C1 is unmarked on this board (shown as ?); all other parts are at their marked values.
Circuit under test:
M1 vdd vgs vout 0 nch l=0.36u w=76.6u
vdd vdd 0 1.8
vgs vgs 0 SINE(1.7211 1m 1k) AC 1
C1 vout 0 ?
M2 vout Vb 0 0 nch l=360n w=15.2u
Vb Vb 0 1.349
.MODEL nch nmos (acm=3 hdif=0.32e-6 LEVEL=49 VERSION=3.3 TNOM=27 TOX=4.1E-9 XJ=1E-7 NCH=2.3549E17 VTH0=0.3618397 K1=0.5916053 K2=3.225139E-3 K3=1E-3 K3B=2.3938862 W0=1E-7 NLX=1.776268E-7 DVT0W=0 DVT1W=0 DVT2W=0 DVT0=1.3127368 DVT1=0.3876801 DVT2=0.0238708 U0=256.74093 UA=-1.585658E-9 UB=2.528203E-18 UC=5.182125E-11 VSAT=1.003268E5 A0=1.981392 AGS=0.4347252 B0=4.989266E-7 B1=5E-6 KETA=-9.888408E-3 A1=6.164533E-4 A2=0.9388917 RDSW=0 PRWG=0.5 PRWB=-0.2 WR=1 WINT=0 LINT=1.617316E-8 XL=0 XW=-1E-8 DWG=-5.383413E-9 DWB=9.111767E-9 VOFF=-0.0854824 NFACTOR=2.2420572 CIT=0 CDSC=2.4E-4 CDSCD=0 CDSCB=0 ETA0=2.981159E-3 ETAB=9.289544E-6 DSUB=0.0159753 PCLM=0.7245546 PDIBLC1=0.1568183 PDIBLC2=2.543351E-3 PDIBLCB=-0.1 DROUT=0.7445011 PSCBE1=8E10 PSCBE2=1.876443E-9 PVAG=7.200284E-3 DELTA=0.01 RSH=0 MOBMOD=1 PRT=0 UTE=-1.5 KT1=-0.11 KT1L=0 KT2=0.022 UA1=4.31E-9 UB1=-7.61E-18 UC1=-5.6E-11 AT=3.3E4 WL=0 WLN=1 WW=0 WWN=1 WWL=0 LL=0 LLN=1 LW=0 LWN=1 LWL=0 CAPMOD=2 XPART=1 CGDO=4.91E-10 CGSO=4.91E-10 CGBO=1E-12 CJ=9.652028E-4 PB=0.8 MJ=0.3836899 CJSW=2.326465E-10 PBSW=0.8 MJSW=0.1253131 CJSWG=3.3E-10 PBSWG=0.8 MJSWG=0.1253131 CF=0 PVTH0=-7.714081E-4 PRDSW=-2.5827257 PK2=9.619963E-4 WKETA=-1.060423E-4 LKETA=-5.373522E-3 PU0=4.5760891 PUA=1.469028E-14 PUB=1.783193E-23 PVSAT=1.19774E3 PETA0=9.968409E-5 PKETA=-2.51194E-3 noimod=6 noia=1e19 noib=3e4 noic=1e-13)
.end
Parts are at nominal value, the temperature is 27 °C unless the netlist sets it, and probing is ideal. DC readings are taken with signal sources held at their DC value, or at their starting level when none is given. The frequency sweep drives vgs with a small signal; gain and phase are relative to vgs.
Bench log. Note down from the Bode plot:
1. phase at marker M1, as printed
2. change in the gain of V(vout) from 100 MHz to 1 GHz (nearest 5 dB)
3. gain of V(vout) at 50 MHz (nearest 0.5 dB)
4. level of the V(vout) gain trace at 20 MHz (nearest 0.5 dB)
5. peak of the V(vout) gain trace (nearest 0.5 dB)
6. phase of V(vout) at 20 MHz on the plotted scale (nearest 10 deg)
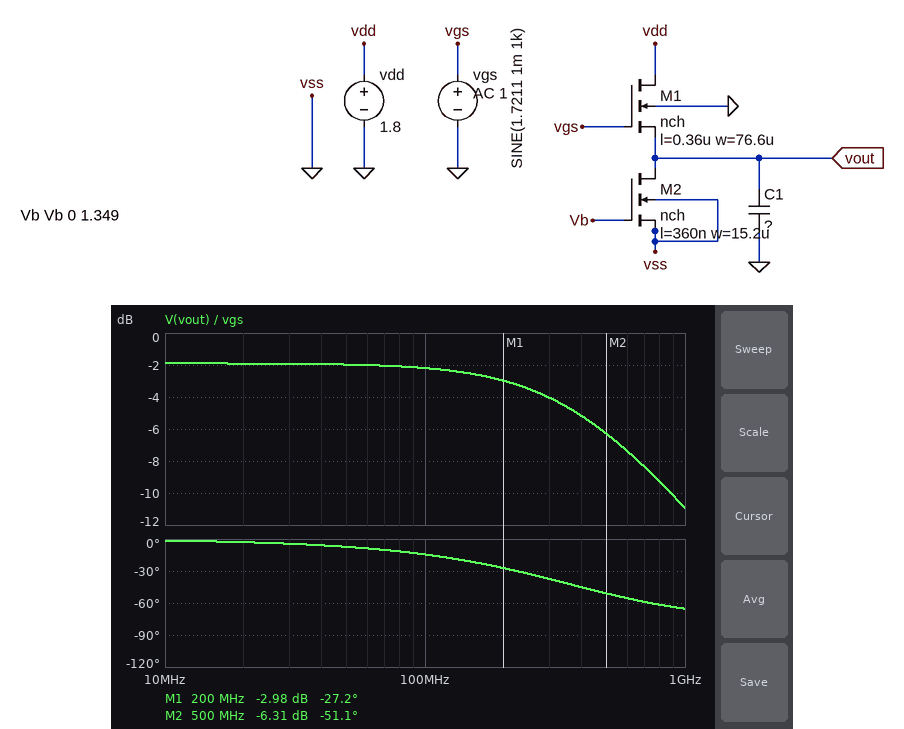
-27.2 deg
-10 dB
-2.0 dB
-2.0 dB
-2.0 dB
0 deg
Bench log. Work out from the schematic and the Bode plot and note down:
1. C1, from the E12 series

8.2 pF
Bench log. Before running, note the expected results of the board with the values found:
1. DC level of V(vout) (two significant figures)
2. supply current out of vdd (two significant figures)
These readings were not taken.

750 mV
3.0 mA
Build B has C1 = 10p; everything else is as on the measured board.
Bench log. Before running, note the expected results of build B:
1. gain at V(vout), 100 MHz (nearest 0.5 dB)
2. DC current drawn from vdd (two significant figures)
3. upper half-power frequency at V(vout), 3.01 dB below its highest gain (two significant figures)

-2.5 dB
3.0 mA
310 MHz
